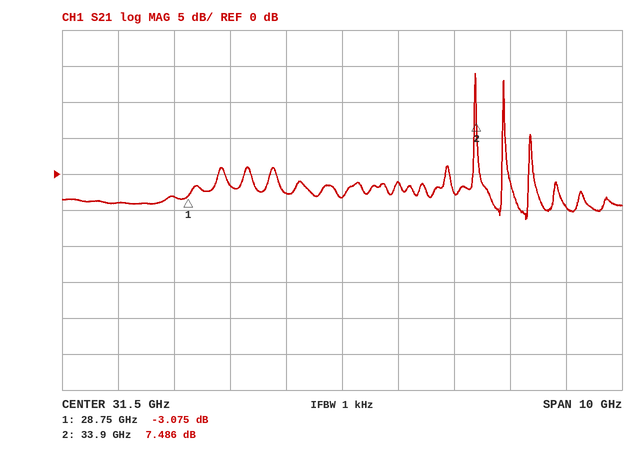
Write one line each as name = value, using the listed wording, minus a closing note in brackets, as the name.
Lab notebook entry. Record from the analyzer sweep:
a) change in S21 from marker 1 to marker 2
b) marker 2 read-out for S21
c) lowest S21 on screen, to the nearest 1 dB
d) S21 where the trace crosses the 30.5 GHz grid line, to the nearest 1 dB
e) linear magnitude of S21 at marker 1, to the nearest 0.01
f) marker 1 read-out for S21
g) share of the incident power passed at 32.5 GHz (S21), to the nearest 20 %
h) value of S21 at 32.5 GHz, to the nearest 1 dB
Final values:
change in S21 from marker 1 to marker 2 = 10.561 dB
marker 2 read-out for S21 = 7.486 dB
lowest S21 on screen, to the nearest 1 dB = -6 dB
S21 where the trace crosses the 30.5 GHz grid line, to the nearest 1 dB = -3 dB
linear magnitude of S21 at marker 1, to the nearest 0.01 = 0.70
marker 1 read-out for S21 = -3.075 dB
share of the incident power passed at 32.5 GHz (S21), to the nearest 20 % = 80 %
value of S21 at 32.5 GHz, to the nearest 1 dB = -1 dB
